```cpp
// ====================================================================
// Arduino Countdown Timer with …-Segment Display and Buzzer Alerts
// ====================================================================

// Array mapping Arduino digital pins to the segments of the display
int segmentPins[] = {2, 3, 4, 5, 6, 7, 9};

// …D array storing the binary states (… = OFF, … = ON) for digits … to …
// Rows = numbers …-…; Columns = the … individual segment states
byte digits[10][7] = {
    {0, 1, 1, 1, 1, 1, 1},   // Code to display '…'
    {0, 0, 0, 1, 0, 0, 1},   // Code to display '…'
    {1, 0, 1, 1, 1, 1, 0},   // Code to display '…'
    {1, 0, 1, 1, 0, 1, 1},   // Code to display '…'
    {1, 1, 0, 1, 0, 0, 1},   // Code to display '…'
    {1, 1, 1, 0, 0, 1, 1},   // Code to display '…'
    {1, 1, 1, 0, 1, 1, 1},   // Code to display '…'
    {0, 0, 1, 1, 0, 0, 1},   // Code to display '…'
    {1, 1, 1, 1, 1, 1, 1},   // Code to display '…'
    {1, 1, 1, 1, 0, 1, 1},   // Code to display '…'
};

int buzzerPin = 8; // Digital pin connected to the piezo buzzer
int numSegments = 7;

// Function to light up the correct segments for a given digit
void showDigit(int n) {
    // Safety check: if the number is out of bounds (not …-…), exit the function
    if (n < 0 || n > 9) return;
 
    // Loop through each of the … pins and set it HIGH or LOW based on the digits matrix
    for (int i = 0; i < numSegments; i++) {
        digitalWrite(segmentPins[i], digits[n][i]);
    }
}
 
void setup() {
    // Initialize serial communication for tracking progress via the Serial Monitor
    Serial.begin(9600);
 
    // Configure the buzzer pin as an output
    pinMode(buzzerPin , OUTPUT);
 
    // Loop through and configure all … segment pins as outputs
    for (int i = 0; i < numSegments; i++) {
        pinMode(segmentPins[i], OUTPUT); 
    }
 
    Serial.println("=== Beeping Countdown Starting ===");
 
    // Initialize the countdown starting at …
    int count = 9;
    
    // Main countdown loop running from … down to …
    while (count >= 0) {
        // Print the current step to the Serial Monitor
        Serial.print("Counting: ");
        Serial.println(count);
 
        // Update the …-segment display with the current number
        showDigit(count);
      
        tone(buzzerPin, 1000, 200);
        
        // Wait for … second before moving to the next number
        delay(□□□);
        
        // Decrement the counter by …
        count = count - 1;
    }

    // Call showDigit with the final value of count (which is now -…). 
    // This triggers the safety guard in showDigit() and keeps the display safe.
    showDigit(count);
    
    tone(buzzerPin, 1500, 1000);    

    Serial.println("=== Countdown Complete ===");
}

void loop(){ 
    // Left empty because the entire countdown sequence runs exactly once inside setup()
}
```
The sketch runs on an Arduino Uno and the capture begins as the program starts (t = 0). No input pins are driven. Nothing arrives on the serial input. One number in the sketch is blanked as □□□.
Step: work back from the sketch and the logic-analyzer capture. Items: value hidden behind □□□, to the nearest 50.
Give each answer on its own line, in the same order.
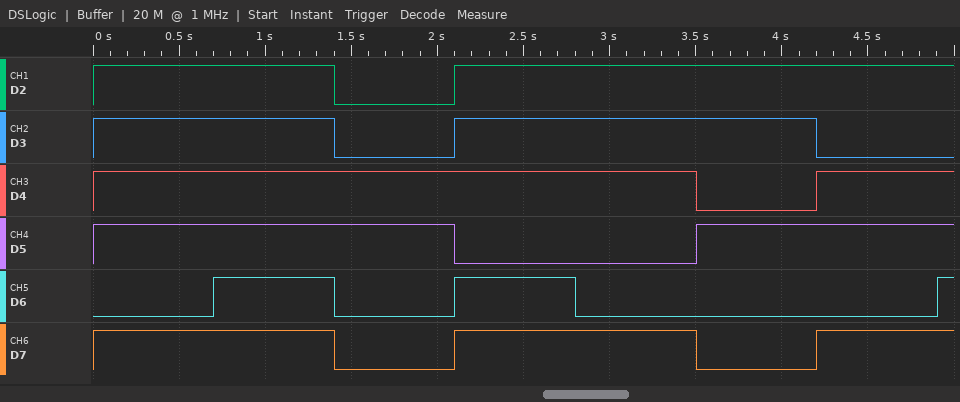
700
